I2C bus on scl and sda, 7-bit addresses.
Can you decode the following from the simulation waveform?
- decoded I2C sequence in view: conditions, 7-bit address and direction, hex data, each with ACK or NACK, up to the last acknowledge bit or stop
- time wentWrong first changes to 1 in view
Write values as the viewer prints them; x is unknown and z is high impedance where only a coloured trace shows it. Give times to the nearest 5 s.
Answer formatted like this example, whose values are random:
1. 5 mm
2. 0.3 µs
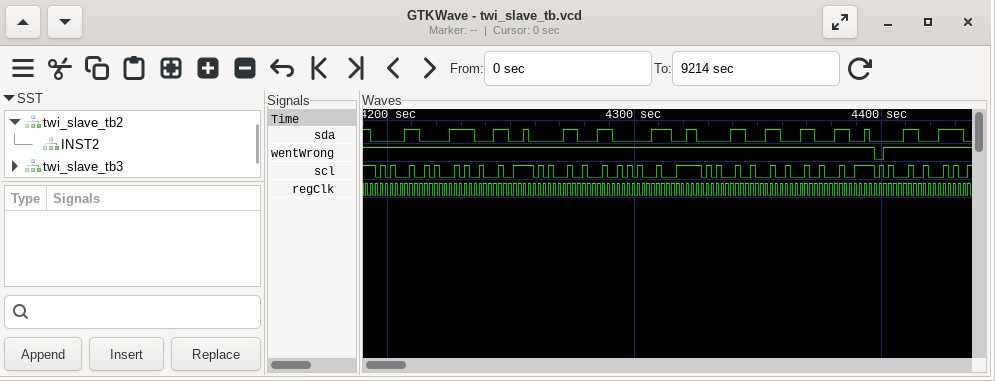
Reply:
1. start, address 13 write NACK, stop, start, address 14 write NACK, stop, start, address 15 write NACK, stop
2. 4400 s
